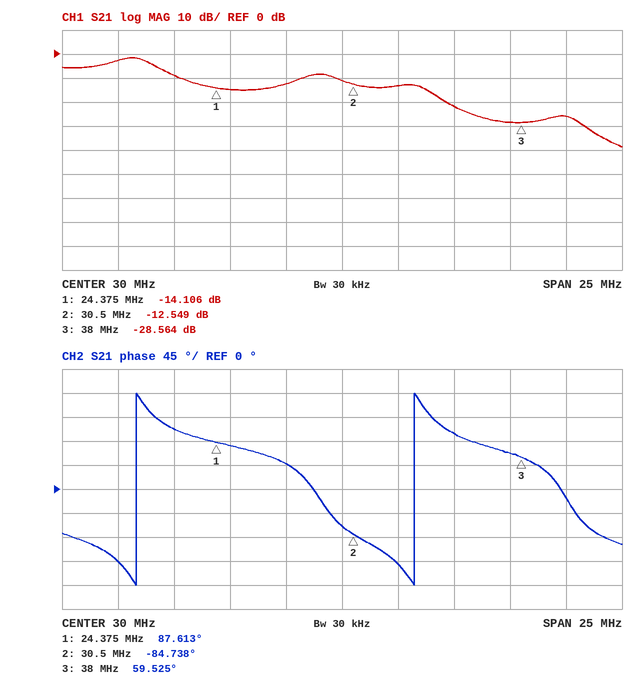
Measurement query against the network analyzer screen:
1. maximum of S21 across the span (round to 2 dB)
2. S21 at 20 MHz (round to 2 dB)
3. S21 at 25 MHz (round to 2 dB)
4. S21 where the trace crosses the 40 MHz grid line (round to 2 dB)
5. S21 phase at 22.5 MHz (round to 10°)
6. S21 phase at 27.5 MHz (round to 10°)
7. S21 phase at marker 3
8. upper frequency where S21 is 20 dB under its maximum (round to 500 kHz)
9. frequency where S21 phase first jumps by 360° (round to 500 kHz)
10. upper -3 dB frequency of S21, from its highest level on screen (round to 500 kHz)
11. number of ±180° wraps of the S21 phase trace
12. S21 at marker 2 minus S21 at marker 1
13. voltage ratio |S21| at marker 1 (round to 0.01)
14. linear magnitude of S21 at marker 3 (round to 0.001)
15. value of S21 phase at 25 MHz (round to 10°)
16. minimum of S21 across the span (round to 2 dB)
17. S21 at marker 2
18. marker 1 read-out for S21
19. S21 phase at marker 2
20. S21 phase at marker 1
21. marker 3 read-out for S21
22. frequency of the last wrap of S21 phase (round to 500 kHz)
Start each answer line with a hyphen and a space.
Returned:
- -2 dB
- -2 dB
- -14 dB
- -26 dB
- 110°
- 50°
- 59.525°
- 35.0 MHz
- 21.0 MHz
- 21.5 MHz
- 2
- 1.557 dB
- 0.20
- 0.037
- 80°
- -38 dB
- -12.549 dB
- -14.106 dB
- -84.738°
- 87.613°
- -28.564 dB
- 33.0 MHz
